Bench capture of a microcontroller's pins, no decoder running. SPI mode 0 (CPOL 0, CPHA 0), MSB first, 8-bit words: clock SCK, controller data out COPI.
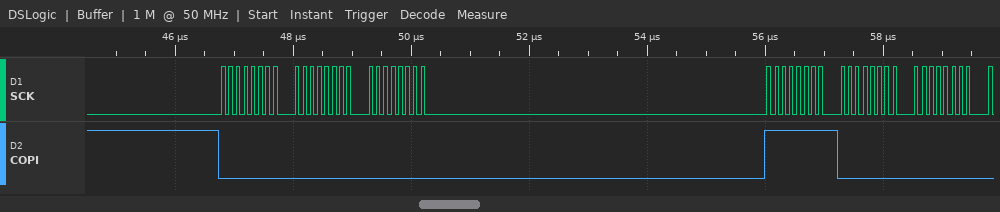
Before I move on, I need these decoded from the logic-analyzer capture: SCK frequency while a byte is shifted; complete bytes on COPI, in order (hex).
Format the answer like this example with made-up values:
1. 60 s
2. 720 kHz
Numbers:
1. 8 MHz
2. 00 00 00 FF 00 00
